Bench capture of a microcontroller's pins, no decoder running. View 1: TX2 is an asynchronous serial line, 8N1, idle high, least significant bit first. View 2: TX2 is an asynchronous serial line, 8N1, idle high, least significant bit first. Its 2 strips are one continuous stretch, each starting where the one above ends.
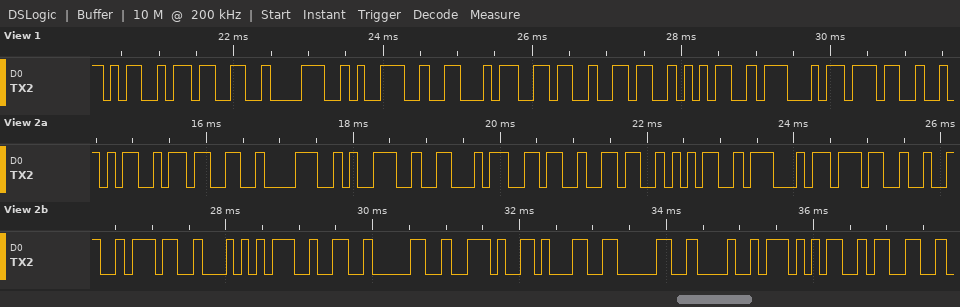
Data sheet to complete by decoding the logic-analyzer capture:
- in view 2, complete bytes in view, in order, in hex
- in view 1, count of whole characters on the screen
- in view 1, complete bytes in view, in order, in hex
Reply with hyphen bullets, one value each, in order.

- 4D 33 38 39 46 36 36 35 47 37 32 37 54 32 30 2E 31 30 48 35 33
- 10
- 4D 33 38 39 46 36 36 35 47 37
